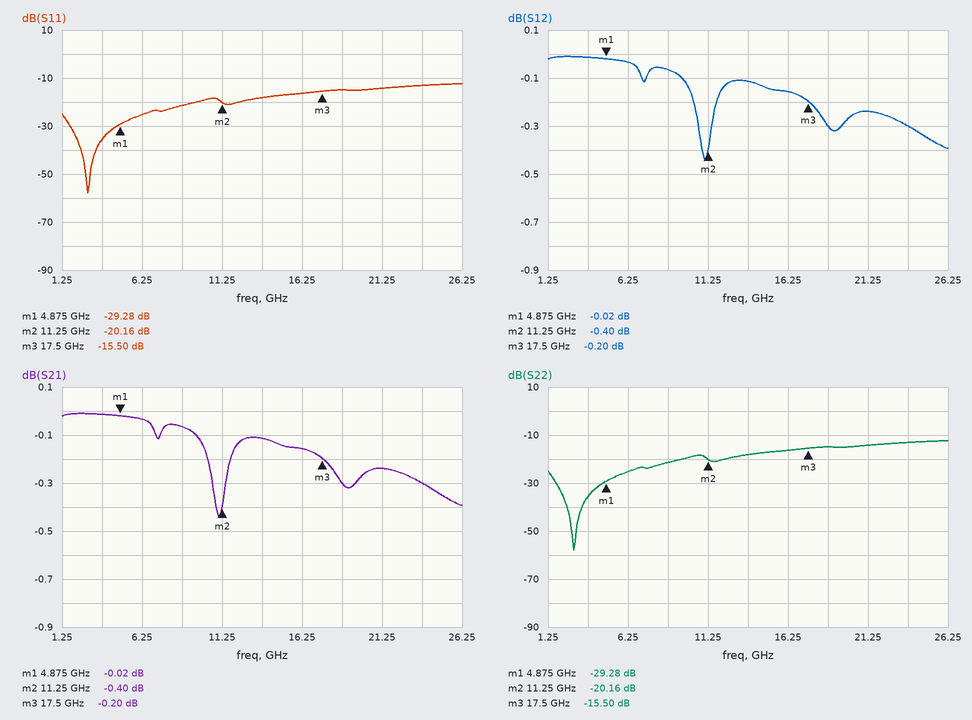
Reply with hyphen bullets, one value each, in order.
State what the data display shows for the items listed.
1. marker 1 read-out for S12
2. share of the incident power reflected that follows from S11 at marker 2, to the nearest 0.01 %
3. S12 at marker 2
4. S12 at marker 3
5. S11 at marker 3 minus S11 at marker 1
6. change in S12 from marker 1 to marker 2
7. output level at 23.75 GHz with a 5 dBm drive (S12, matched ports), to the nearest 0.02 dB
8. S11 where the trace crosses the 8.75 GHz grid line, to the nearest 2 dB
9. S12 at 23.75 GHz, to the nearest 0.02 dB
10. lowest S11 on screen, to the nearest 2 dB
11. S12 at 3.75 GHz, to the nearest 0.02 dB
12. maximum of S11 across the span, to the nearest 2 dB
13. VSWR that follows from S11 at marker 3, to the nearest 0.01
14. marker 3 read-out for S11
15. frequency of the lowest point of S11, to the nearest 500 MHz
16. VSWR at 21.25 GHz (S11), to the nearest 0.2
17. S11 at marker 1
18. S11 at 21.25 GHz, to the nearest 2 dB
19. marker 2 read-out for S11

- -0.02 dB
- 0.96 %
- -0.40 dB
- -0.20 dB
- 13.78 dB
- -0.38 dB
- 4.70 dBm
- -22 dB
- -0.30 dB
- -58 dB
- -0.02 dB
- -12 dB
- 1.40
- -15.50 dB
- 3.0 GHz
- 1.4
- -29.28 dB
- -14 dB
- -20.16 dB
